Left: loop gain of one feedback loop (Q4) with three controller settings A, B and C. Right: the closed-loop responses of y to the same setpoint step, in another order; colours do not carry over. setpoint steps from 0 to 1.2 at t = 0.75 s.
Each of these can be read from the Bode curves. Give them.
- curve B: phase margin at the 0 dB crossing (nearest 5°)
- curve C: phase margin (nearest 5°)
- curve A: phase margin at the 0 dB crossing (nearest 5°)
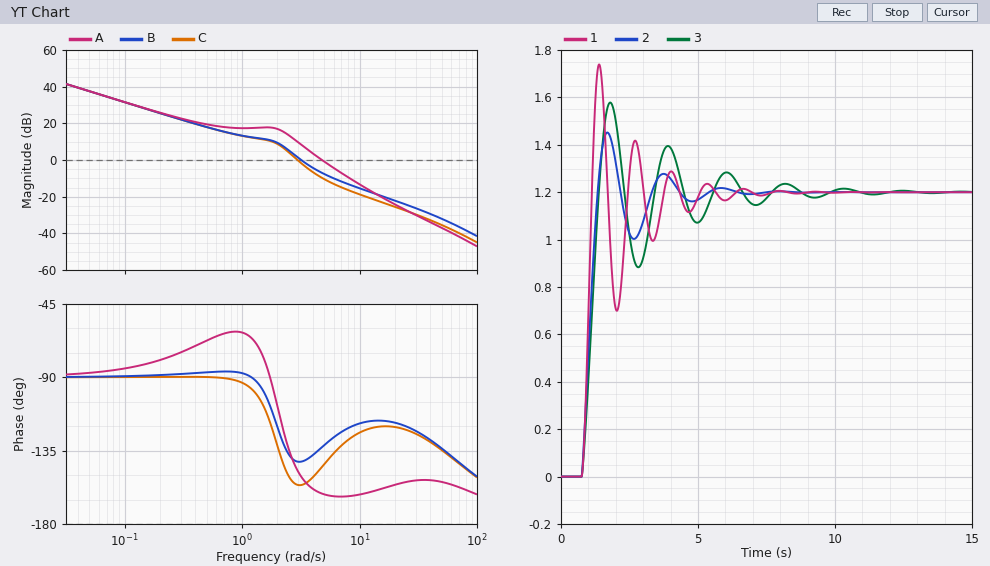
40°
25°
20°
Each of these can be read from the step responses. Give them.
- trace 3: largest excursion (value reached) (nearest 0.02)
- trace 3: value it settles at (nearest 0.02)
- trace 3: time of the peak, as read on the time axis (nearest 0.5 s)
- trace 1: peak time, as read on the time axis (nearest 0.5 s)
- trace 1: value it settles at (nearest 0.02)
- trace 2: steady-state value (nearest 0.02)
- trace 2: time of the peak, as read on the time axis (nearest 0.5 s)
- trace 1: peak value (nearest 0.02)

1.58
1.20
2.0 s
1.5 s
1.20
1.20
1.5 s
1.74
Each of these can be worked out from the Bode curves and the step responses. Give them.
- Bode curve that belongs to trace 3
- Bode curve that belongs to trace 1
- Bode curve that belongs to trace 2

C
A
B
